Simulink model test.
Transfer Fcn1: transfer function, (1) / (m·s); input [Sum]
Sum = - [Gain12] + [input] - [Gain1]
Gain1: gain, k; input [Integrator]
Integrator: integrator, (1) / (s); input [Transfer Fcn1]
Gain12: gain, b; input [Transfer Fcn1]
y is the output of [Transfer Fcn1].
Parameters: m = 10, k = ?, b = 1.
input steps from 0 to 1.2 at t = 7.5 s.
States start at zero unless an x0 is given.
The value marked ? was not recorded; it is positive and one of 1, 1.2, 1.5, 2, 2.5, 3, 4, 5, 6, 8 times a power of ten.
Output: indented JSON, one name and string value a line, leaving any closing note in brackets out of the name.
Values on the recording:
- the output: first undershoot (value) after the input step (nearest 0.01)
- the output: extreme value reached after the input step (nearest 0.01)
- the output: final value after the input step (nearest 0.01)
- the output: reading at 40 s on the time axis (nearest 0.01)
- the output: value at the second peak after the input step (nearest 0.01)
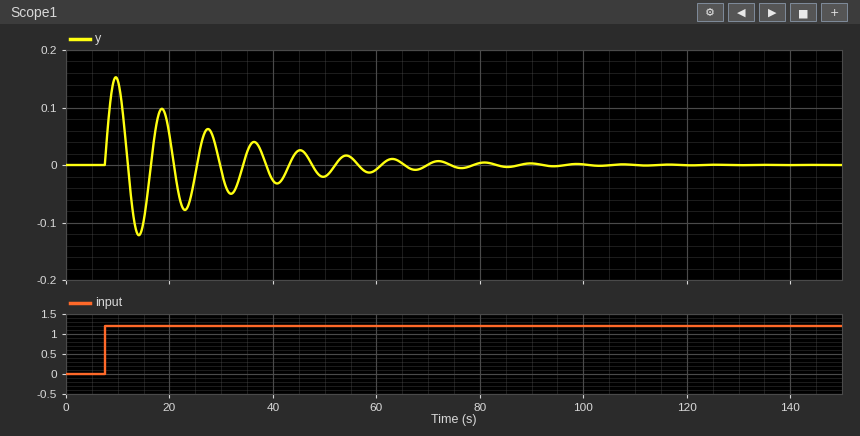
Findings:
{
  "the output: first undershoot (value) after the input step": "-0.12",
  "the output: extreme value reached after the input step": "0.15",
  "the output: final value after the input step": "0.00",
  "the output: reading at 40 s on the time axis": "-0.03",
  "the output: value at the second peak after the input step": "0.10"
}
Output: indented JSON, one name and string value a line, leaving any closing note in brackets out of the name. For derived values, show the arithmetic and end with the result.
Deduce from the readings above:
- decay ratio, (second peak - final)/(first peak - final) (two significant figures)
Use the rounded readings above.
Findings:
{
  "decay ratio, (second peak - final)/(first peak - final)": "(0.1 - 0) / (0.15 - 0) = 0.67"
}
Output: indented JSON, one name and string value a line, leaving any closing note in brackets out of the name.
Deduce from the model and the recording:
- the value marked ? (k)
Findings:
{
  "the value marked ?": "5"
}
